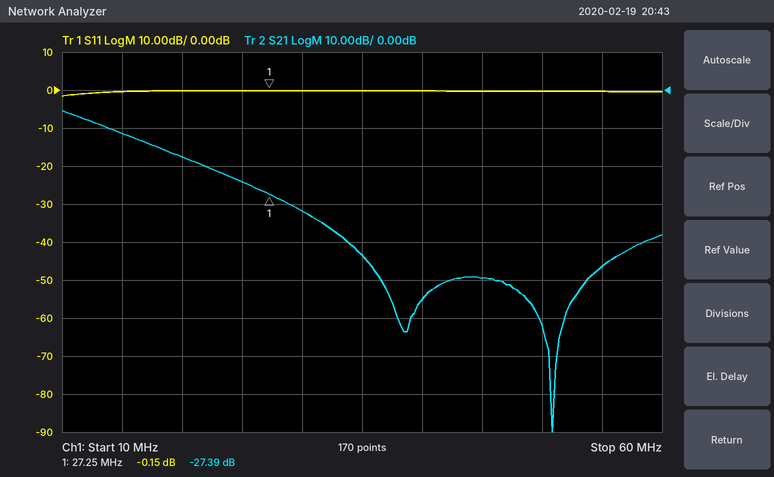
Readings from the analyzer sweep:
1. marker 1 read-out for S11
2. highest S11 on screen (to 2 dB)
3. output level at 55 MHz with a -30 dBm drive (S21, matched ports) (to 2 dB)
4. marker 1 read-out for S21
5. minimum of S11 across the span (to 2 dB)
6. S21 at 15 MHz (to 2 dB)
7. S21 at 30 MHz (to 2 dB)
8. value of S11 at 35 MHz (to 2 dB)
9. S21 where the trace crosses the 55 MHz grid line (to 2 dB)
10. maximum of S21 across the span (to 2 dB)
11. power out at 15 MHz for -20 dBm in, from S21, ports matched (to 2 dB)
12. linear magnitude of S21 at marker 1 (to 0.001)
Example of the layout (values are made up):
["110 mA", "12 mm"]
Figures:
["-0.15 dB", "0 dB", "-76 dBm", "-27.39 dB", "-2 dB", "-12 dB", "-32 dB", "0 dB", "-46 dB", "-6 dB", "-32 dBm", "0.043"]
